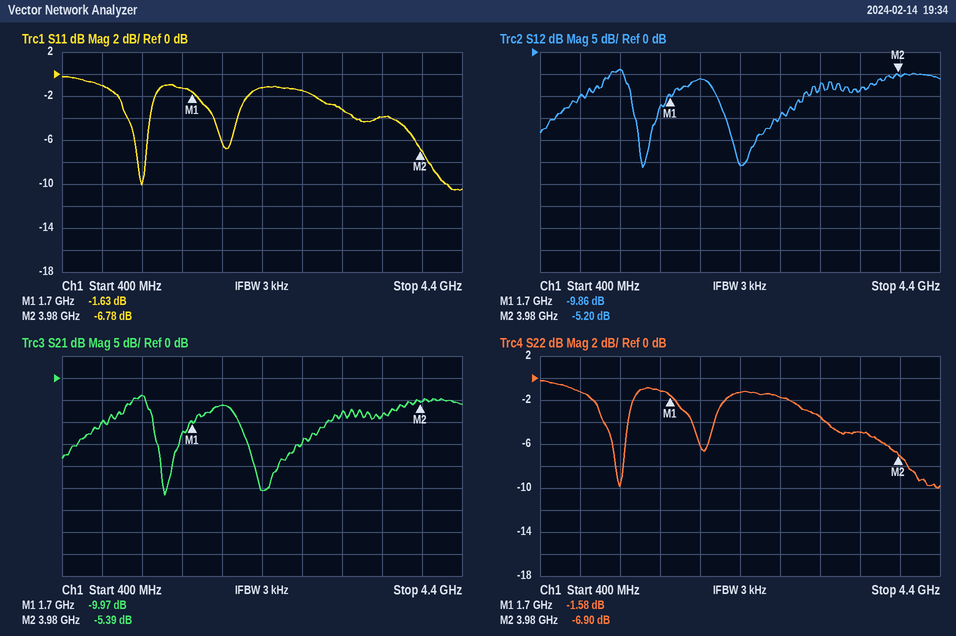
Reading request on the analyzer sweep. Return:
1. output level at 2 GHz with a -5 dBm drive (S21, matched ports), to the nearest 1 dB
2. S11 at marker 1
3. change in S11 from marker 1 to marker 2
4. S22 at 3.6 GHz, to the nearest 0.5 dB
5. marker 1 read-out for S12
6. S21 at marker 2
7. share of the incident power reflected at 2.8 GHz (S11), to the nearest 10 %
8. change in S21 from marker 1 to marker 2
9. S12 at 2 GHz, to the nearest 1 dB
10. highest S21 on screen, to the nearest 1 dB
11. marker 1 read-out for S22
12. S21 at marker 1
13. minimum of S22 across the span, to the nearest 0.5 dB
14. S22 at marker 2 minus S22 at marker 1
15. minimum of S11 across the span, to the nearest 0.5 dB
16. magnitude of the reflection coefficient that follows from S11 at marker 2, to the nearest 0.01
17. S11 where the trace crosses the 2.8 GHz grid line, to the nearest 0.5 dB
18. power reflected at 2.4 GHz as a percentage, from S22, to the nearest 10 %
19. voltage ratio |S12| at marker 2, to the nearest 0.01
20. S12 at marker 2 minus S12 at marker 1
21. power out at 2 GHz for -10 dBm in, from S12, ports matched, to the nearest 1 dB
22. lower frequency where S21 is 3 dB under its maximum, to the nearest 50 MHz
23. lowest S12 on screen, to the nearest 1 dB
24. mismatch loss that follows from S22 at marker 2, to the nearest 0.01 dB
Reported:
-11 dBm
-1.63 dB
-5.15 dB
-5.0 dB
-9.86 dB
-5.39 dB
70 %
4.58 dB
-6 dB
-4 dB
-1.58 dB
-9.97 dB
-10.0 dB
-5.32 dB
-10.5 dB
0.46
-1.5 dB
70 %
0.55
4.66 dB
-16 dBm
1.05 GHz
-26 dB
0.99 dB
